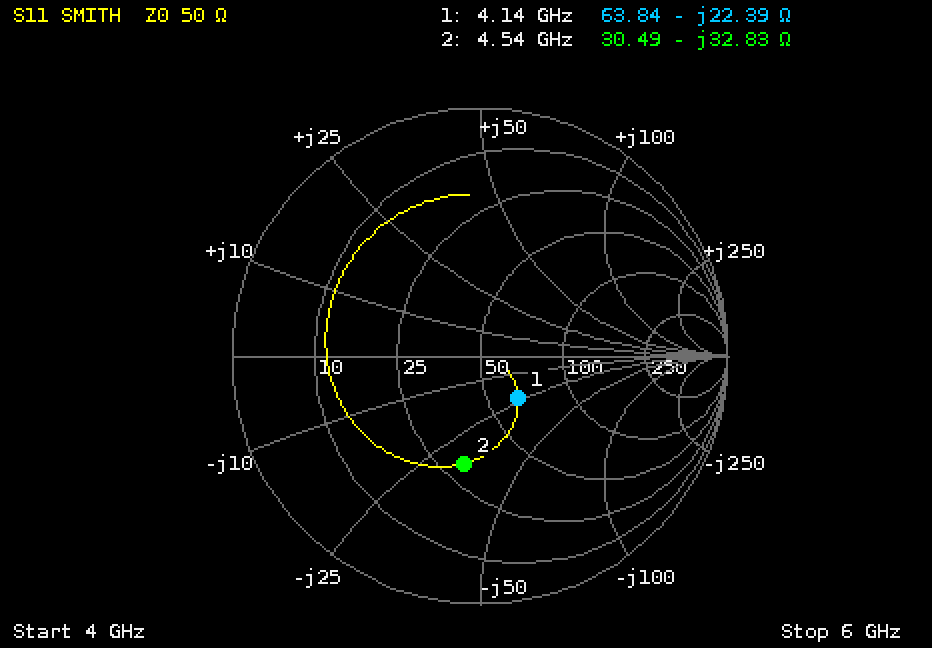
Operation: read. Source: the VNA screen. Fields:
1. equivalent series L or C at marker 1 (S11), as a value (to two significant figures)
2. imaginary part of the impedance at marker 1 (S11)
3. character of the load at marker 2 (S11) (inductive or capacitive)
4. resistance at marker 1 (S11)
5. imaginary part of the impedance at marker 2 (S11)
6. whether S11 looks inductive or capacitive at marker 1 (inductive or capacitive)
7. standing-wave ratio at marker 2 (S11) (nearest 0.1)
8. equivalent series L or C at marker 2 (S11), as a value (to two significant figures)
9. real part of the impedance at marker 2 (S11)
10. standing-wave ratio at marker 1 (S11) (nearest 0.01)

1.7 pF
-22.39 Ω
capacitive
63.84 Ω
-32.83 Ω
capacitive
2.6
1.1 pF
30.49 Ω
1.59
